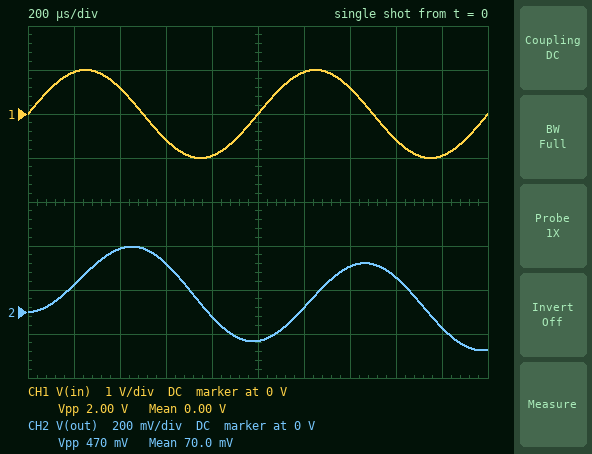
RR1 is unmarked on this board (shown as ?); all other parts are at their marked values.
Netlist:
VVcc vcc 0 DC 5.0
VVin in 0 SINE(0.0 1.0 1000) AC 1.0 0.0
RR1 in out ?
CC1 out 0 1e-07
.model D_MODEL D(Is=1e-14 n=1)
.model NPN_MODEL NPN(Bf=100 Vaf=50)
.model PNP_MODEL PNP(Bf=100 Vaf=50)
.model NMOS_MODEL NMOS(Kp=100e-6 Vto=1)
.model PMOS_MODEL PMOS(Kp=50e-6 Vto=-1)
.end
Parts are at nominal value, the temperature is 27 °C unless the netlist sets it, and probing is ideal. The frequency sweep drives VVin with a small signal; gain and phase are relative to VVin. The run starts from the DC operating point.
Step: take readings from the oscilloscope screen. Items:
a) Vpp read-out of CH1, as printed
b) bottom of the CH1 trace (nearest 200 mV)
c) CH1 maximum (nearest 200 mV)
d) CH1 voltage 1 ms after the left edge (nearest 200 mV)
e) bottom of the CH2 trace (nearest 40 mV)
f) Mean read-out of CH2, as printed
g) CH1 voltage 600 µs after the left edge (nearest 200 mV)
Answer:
2.00 V
-1.0 V
1.0 V
0 V
-160 mV
70.0 mV
-600 mV
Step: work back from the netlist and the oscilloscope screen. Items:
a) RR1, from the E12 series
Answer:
8.2 kΩ
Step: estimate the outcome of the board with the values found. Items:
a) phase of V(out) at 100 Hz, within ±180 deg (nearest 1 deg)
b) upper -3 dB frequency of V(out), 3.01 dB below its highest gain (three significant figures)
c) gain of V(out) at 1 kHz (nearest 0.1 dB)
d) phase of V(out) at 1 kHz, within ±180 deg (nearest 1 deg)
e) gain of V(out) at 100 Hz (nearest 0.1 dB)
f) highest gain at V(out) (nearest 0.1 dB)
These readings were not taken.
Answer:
-27 deg
194 Hz
-14.4 dB
-79 deg
-1.0 dB
0 dB
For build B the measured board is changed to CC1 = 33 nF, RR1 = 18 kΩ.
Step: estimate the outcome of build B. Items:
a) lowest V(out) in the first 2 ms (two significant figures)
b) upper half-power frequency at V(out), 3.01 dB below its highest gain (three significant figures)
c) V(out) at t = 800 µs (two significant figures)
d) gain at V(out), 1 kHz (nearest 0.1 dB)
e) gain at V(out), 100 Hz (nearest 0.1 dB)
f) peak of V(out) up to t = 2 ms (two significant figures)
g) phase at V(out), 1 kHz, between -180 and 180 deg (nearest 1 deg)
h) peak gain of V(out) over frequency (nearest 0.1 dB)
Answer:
-250 mV
268 Hz
-76 mV
-11.7 dB
-0.6 dB
380 mV
-75 deg
0 dB
